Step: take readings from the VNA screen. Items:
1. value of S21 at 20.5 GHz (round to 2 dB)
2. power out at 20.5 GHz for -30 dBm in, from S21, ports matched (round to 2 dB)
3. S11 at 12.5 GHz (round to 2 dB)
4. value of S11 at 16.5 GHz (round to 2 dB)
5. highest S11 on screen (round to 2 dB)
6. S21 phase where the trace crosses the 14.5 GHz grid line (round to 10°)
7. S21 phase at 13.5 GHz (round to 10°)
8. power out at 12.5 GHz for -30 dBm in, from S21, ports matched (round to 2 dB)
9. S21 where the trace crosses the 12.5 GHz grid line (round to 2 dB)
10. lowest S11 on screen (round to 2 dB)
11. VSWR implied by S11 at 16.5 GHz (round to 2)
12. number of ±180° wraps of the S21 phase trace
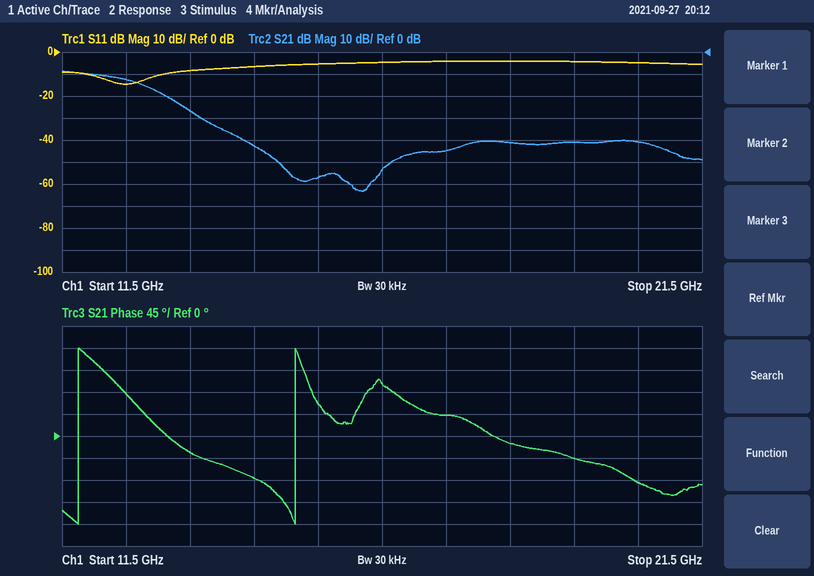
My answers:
-40 dB
-70 dBm
-14 dB
-4 dB
-4 dB
-90°
-30°
-42 dBm
-12 dB
-14 dB
4
2
